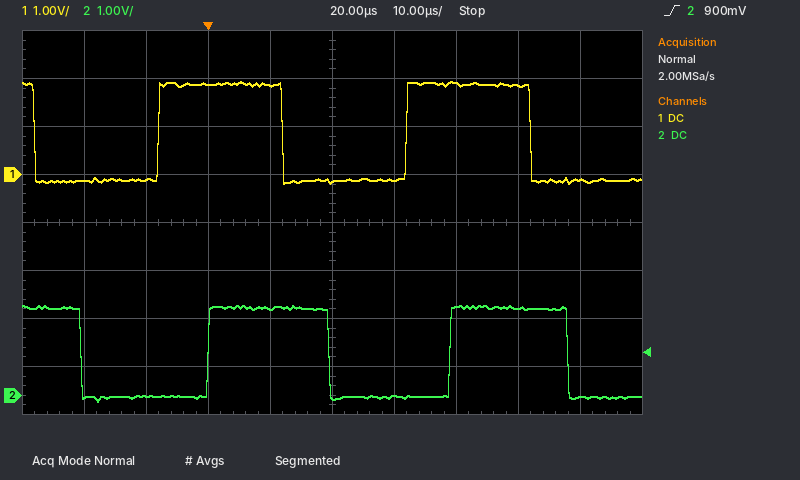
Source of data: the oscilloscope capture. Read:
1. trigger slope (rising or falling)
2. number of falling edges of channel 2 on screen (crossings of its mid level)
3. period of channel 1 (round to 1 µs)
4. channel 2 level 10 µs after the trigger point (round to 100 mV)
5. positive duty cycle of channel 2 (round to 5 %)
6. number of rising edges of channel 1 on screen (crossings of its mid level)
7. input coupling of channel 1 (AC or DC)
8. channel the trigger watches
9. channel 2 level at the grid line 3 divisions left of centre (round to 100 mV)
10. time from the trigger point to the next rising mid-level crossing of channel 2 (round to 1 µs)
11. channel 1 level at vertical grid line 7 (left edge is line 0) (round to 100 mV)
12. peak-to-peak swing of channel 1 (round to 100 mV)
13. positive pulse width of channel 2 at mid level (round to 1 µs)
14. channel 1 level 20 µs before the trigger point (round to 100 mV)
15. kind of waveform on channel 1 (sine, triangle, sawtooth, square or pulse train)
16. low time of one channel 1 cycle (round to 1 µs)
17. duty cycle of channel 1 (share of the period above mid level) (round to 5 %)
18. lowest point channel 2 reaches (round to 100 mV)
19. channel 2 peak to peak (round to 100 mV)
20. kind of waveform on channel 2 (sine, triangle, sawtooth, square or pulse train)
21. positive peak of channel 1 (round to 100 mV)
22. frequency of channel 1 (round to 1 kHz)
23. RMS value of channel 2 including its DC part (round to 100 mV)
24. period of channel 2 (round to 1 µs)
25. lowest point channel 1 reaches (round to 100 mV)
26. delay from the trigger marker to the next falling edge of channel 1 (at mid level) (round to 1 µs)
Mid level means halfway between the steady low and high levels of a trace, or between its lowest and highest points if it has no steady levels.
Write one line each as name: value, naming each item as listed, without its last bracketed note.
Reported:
trigger slope: rising
number of falling edges of channel 2 on screen: 3
period of channel 1: 40 µs
channel 2 level 10 µs after the trigger point: 1.8 V
positive duty cycle of channel 2: 50 %
number of rising edges of channel 1 on screen: 2
input coupling of channel 1: DC
channel the trigger watches: channel 2
channel 2 level at the grid line 3 divisions left of centre: 0.0 V
time from the trigger point to the next rising mid-level crossing of channel 2: 39 µs
channel 1 level at vertical grid line 7 (left edge is line 0): 1.9 V
peak-to-peak swing of channel 1: 2.1 V
positive pulse width of channel 2 at mid level: 19 µs
channel 1 level 20 µs before the trigger point: -100 mV
kind of waveform on channel 1: square
low time of one channel 1 cycle: 20 µs
duty cycle of channel 1 (share of the period above mid level): 50 %
lowest point channel 2 reaches: -100 mV
channel 2 peak to peak: 2.0 V
kind of waveform on channel 2: square
positive peak of channel 1: 1.9 V
frequency of channel 1: 25 kHz
RMS value of channel 2 including its DC part: 1.3 V
period of channel 2: 39 µs
lowest point channel 1 reaches: -200 mV
delay from the trigger marker to the next falling edge of channel 1 (at mid level): 12 µs
